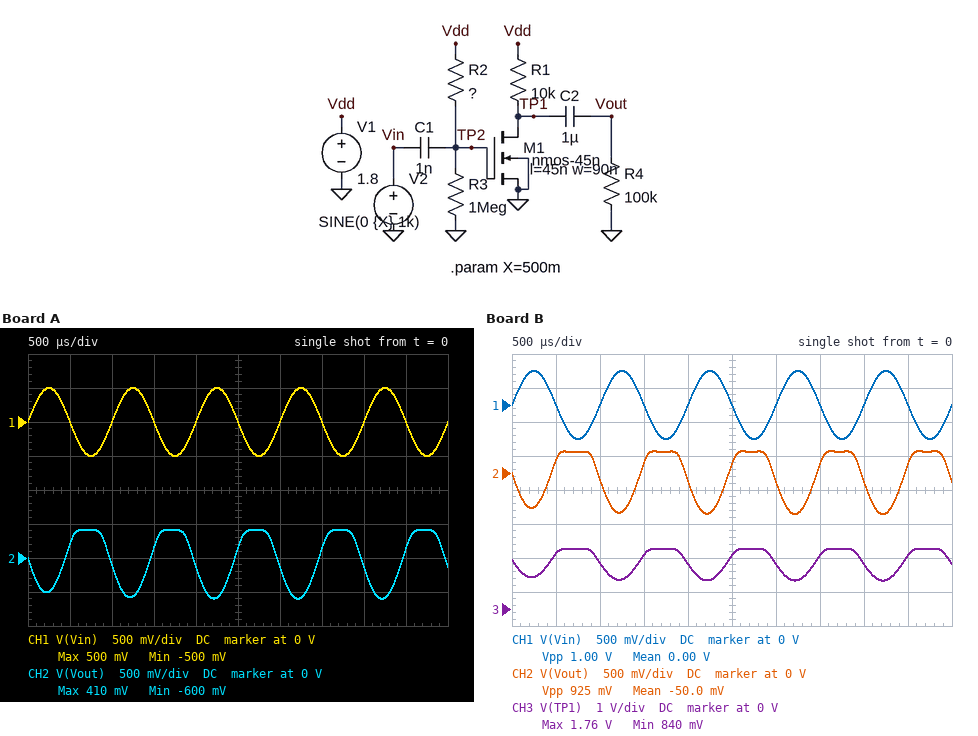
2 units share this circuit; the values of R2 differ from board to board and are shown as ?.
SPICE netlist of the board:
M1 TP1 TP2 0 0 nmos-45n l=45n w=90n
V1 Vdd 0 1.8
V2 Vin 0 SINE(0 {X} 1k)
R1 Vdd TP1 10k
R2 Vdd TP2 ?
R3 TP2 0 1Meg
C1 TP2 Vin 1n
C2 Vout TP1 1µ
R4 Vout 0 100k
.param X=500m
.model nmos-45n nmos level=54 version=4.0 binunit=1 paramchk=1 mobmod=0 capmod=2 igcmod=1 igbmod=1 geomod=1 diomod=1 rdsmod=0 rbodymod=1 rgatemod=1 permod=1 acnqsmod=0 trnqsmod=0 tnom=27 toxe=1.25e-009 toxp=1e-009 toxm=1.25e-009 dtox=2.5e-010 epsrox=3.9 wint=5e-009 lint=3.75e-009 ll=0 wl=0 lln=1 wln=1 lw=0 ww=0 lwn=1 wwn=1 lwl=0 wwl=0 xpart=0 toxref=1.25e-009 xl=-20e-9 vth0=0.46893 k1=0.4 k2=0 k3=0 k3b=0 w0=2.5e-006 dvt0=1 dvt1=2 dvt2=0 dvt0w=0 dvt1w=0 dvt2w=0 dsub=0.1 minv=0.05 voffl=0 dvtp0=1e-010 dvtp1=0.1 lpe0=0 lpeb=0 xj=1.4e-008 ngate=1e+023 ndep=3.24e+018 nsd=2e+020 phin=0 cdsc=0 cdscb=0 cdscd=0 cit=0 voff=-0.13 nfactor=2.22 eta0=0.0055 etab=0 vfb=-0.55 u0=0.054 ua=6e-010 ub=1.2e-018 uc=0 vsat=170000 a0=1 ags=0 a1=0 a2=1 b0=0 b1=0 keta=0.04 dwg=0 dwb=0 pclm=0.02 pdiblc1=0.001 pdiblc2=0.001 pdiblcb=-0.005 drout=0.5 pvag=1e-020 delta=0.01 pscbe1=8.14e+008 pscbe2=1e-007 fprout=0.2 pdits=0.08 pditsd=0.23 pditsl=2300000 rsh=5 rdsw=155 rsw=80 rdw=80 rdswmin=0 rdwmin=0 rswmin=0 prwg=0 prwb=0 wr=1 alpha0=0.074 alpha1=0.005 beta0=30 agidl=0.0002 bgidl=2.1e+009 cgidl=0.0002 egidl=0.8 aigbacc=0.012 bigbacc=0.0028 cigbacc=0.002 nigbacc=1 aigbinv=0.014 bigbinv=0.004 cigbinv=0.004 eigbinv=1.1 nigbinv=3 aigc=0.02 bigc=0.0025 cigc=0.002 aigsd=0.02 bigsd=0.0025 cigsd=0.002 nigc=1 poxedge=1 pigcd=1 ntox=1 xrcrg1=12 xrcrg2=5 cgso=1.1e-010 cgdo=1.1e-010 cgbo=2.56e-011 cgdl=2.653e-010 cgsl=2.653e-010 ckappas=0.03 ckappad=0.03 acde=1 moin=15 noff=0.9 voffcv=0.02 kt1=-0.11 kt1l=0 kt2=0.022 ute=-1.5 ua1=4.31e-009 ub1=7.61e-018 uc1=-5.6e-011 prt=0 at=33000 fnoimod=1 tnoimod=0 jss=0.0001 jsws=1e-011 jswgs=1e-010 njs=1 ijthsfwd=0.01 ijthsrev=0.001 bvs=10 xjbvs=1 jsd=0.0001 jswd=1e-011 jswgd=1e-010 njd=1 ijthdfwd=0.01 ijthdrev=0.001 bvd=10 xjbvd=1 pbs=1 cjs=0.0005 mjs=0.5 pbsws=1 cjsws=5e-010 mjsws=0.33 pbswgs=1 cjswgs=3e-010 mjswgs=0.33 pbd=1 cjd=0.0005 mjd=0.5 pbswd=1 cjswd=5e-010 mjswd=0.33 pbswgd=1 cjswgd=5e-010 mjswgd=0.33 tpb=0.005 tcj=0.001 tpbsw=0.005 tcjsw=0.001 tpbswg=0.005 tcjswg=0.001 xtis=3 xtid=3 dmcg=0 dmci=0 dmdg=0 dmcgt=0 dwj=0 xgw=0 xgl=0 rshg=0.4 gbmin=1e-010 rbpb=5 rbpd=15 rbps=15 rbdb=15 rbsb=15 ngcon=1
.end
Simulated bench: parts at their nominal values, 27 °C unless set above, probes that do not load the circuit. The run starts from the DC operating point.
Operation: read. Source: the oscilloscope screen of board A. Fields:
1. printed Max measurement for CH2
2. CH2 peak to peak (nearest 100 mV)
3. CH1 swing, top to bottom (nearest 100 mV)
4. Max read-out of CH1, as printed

410 mV
1.0 V
1.0 V
500 mV
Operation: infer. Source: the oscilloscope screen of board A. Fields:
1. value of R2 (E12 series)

2.2 MΩ
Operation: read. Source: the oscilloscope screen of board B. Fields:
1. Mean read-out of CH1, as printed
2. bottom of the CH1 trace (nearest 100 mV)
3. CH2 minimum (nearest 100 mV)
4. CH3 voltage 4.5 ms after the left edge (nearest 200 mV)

0.00 V
-500 mV
-600 mV
1.6 V
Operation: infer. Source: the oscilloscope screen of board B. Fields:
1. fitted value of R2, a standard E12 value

2.7 MΩ
